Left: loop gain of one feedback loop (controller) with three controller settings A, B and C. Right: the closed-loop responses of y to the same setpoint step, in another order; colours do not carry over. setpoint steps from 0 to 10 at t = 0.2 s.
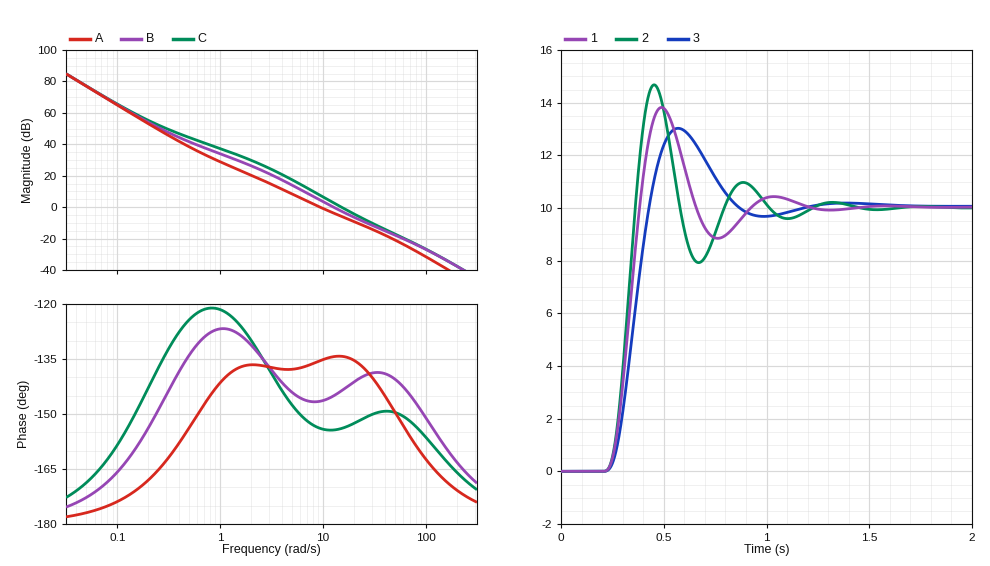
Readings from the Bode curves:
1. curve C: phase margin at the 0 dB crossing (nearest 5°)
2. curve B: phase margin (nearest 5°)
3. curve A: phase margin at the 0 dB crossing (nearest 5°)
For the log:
25°
35°
45°
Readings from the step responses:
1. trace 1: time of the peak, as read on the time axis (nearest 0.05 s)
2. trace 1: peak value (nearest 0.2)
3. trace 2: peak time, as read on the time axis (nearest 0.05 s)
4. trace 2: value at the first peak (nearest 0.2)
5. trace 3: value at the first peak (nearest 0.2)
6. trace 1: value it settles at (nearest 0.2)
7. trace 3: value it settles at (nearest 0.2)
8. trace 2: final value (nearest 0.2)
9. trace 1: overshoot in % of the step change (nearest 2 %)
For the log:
0.50 s
13.8
0.45 s
14.6
13.0
10.0
10.0
10.0
38 %
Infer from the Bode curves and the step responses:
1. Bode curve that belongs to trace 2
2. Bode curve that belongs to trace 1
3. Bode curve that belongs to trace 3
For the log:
C
B
A
